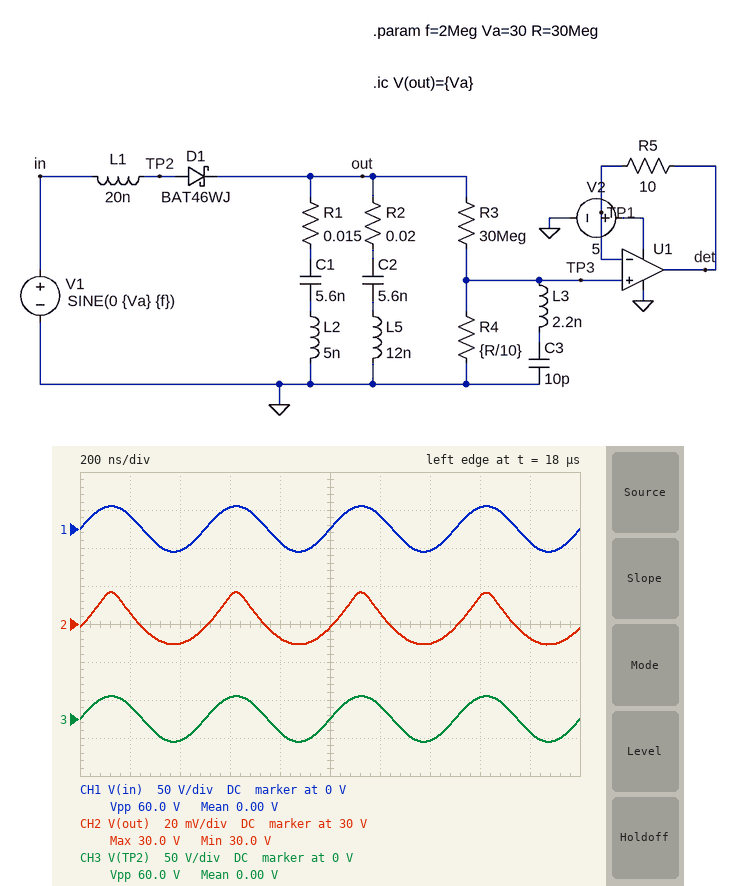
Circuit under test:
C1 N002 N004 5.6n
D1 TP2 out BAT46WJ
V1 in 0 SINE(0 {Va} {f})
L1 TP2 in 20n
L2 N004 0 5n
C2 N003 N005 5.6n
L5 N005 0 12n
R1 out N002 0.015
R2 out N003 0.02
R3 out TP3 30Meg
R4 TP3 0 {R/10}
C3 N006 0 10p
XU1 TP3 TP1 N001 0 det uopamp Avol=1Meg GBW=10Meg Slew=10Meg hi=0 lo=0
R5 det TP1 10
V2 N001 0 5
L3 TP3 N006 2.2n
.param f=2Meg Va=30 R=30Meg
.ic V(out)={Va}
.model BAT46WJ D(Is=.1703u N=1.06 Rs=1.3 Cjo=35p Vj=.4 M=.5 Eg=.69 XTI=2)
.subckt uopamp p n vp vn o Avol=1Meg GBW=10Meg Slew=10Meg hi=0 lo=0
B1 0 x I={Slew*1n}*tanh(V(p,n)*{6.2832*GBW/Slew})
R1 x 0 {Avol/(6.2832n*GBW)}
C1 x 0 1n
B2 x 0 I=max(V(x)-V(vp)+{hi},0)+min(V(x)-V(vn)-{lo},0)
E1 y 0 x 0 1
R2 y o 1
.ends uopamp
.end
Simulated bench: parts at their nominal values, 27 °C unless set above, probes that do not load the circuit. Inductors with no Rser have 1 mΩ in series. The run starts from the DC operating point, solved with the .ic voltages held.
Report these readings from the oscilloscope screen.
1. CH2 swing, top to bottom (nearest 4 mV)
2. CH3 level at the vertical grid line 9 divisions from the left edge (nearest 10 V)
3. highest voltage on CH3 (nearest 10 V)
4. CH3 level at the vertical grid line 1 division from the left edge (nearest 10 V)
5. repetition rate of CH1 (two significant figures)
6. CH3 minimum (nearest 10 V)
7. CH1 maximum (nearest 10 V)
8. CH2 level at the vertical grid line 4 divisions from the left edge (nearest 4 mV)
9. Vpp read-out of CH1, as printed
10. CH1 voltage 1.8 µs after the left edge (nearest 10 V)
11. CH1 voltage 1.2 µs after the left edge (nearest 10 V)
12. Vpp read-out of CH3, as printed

28 mV
-20 V
30 V
20 V
2.0 MHz
-30 V
30 V
29.992 V
60.0 V
-20 V
20 V
60.0 V
